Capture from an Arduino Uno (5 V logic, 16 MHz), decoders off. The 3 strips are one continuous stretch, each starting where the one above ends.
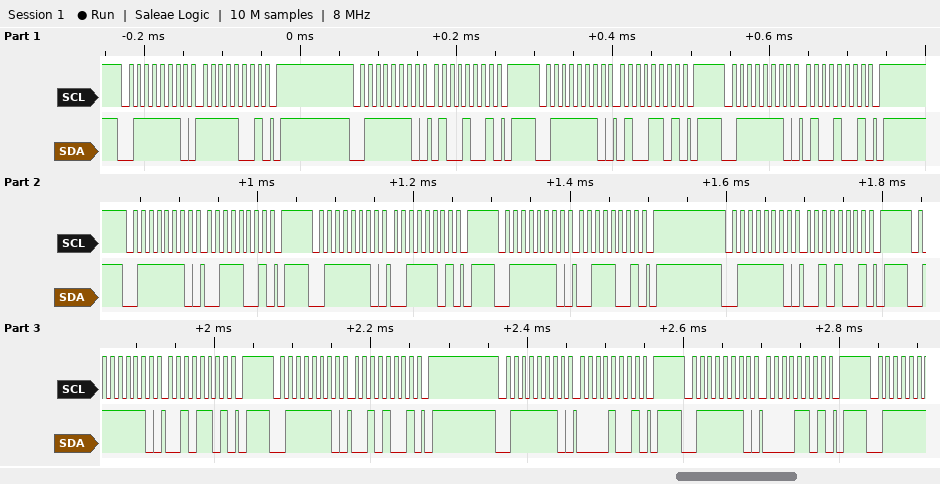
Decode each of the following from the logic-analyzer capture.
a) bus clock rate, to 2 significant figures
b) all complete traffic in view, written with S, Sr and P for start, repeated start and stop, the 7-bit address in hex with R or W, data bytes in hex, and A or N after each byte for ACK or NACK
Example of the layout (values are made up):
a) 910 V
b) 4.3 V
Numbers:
a) 100 kHz
b) S 3FW A F9 A P S 3FW A 49 A P S 3FW A 4D A P S 3FW A 49 A P S 3FW A 39 A P S 3FW A 3D A P S 3FW A 39 A P S 3FW A 29 A P S 3FW A 2D A P S 3FW A 29 A P S 3FW A 09 A P S 3FW A 0D A P
